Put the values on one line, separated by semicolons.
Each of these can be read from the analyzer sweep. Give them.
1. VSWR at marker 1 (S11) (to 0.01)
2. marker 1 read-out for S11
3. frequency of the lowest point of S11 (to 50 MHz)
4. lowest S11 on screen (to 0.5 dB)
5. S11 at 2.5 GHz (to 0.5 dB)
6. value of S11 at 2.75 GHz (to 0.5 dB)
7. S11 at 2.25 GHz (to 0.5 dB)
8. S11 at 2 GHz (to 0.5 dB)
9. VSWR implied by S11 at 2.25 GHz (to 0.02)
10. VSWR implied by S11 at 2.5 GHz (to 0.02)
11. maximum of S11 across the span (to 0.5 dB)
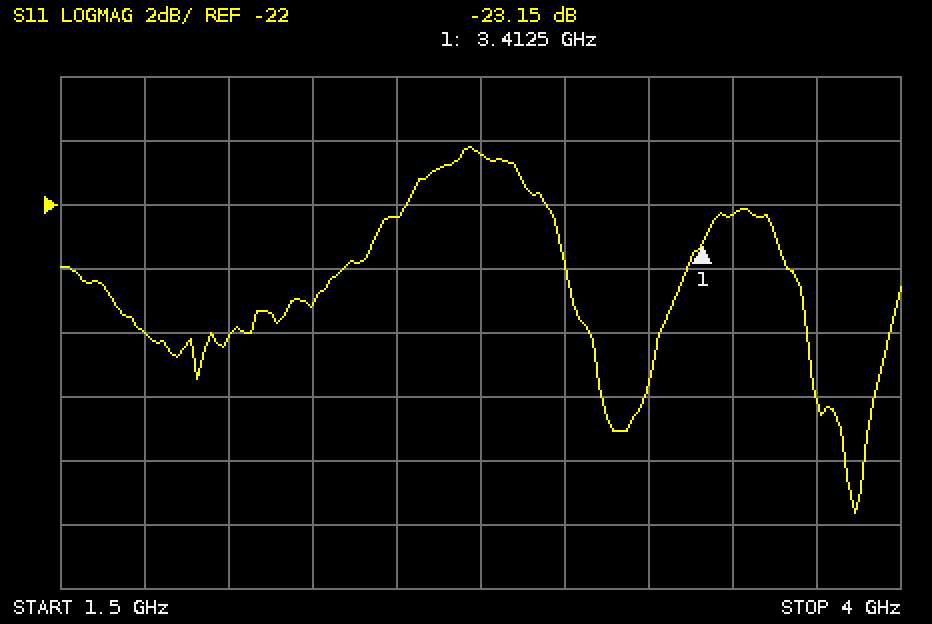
1.15; -23.15 dB; 3.85 GHz; -31.5 dB; -22.5 dB; -20.5 dB; -25.0 dB; -26.0 dB; 1.12; 1.16; -20.0 dB
